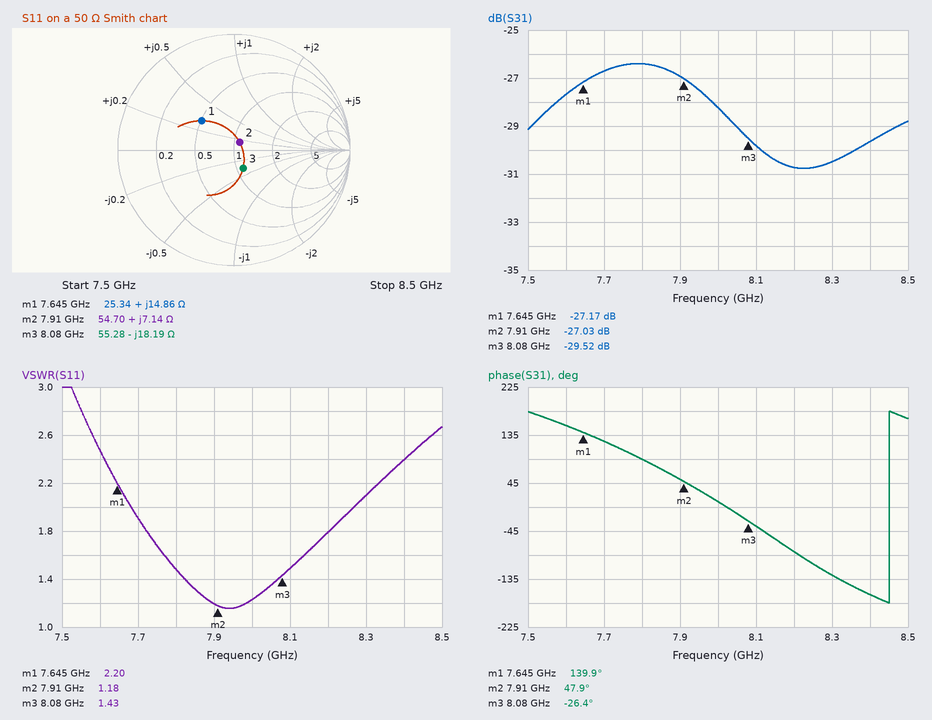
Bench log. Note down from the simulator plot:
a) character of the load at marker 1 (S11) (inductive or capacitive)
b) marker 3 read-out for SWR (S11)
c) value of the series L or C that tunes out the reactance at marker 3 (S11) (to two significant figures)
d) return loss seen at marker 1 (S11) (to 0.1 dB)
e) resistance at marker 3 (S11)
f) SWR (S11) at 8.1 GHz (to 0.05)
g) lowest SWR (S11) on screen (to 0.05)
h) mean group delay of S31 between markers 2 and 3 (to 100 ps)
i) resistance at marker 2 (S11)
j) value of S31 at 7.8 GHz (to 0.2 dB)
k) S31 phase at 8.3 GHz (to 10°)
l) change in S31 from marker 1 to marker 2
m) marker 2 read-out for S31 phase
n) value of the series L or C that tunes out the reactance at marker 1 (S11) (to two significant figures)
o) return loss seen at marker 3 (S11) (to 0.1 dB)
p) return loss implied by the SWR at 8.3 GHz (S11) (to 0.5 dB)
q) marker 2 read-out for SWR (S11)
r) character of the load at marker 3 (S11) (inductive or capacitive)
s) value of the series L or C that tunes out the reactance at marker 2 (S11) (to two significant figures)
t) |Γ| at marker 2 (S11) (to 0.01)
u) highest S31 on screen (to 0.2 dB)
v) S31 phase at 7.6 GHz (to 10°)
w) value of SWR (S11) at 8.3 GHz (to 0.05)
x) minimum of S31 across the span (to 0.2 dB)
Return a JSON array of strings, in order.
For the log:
["inductive", "1.43", "360 pH", "8.5 dB", "55.28 Ω", "1.50", "1.15", "1.2 ns", "54.70 Ω", "-26.4 dB", "-130°", "0.14 dB", "47.9°", "1.4 pF", "15.0 dB", "9.0 dB", "1.18", "capacitive", "2.8 pF", "0.08", "-26.4 dB", "150°", "2.10", "-30.8 dB"]
